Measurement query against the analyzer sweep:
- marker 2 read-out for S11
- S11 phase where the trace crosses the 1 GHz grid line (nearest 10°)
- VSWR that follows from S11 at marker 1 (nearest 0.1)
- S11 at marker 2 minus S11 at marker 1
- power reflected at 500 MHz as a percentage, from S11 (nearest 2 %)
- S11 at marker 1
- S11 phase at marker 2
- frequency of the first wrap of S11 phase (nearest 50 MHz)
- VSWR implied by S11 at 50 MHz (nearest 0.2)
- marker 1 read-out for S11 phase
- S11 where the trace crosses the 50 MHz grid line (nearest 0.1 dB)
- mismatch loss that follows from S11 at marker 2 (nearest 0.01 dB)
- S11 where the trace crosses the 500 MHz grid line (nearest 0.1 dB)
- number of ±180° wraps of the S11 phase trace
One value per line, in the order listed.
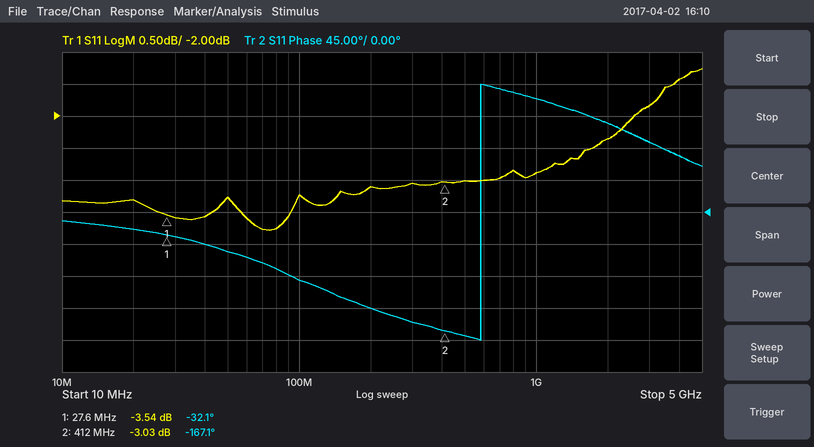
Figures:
-3.03 dB
160°
5.0
0.51 dB
50 %
-3.54 dB
-167.1°
600 MHz
5.4
-32.1°
-3.3 dB
2.99 dB
-3.0 dB
1
